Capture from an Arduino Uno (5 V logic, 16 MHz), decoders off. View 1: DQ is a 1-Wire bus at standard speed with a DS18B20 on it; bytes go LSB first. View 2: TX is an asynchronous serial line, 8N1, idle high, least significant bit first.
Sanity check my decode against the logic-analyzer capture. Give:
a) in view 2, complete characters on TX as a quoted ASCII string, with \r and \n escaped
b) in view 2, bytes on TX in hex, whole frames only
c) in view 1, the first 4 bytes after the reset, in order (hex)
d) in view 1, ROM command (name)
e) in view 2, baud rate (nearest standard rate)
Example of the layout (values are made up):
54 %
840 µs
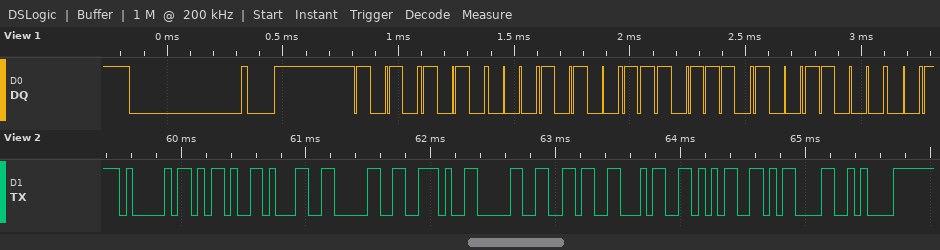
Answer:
"A-10.0645\r\n"
41 2D 31 30 2E 30 36 34 35 0D 0A
55 28 77 19
Match ROM
19200 baud
